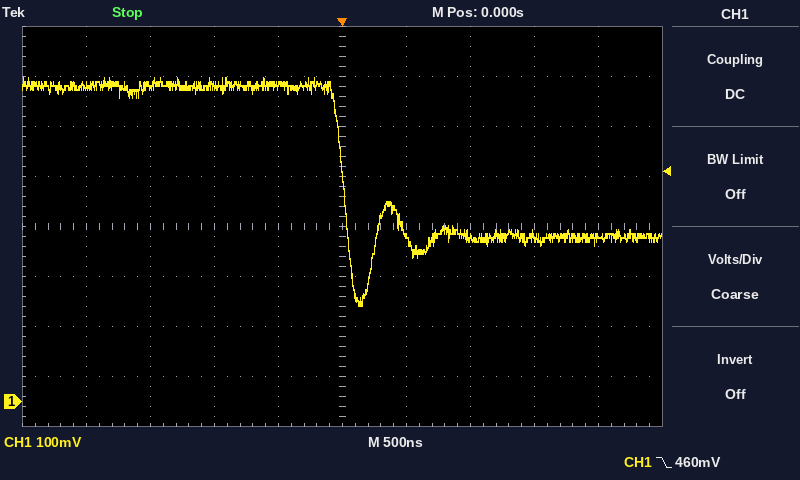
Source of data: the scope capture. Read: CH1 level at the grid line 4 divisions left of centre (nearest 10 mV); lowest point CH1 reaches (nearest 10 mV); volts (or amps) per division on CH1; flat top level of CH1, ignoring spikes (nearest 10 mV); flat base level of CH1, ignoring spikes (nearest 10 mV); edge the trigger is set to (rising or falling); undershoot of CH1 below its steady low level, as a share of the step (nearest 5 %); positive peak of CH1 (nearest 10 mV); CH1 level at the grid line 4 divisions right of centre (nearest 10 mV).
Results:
630 mV
190 mV
100 mV
630 mV
330 mV
falling
45 %
650 mV
330 mV
